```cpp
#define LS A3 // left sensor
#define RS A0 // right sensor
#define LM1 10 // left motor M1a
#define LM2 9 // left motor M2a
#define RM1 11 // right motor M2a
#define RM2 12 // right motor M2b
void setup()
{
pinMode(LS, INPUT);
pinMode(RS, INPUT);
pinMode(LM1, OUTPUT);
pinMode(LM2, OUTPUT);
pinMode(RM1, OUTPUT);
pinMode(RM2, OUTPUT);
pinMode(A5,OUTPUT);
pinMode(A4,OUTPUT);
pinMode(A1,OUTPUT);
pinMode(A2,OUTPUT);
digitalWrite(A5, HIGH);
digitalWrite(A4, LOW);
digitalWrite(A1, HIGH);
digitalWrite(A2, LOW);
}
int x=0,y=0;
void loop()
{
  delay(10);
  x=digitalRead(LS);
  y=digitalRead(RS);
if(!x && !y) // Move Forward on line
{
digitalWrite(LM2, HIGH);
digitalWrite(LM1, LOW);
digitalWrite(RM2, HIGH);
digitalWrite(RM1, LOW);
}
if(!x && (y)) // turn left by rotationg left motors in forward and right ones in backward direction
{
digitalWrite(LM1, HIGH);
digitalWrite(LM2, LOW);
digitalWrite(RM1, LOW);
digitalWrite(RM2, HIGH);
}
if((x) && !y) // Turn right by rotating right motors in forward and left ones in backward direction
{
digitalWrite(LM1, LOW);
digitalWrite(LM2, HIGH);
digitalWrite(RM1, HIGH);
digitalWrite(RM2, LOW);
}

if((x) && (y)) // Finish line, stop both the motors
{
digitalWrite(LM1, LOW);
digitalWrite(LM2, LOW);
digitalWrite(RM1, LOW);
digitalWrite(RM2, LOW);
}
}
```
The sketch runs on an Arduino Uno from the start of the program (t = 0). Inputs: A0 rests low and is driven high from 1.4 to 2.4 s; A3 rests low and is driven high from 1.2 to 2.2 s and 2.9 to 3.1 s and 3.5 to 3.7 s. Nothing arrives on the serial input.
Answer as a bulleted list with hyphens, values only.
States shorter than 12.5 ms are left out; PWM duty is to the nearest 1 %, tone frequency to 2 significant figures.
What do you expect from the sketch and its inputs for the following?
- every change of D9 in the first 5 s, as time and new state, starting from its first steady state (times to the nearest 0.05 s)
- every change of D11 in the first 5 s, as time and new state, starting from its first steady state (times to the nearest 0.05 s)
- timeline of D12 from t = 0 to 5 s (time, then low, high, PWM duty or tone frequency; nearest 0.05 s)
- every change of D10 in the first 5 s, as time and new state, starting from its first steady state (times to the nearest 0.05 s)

- 0 s high; 1.4 s low; 2.4 s high
- 0 s low; 1.2 s high; 1.4 s low; 2.9 s high; 3.1 s low; 3.5 s high; 3.7 s low
- 0 s high; 1.2 s low; 2.2 s high; 2.9 s low; 3.1 s high; 3.5 s low; 3.7 s high
- 0 s low; 2.2 s high; 2.4 s low
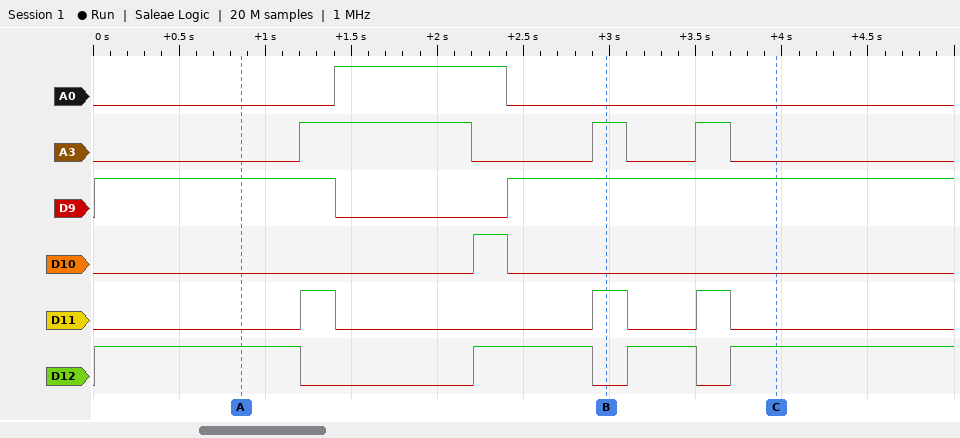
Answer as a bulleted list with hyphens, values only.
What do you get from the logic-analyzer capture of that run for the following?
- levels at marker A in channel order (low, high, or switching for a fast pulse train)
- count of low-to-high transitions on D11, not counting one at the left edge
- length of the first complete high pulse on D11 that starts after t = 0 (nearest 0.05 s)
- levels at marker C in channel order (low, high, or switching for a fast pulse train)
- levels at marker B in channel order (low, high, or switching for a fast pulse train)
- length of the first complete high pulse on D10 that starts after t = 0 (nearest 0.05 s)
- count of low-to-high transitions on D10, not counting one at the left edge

- A0 low, A3 low, D9 high, D10 low, D11 low, D12 high
- 3
- 0.20 s
- A0 low, A3 low, D9 high, D10 low, D11 low, D12 high
- A0 low, A3 high, D9 high, D10 low, D11 high, D12 low
- 0.20 s
- 1
